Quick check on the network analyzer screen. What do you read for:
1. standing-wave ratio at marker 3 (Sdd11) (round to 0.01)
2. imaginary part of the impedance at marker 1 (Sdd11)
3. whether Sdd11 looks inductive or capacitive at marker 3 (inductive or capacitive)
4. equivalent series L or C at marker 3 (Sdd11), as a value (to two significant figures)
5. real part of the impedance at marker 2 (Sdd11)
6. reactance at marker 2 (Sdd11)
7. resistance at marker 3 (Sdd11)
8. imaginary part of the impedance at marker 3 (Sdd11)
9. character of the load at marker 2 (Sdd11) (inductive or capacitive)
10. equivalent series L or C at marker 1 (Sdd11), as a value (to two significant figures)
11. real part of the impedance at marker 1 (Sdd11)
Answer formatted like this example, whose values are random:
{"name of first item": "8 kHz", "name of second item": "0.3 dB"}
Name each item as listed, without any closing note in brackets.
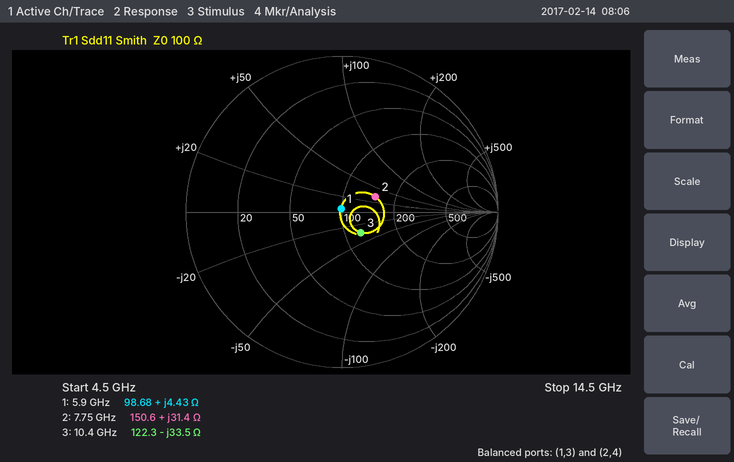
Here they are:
{"standing-wave ratio at marker 3 (Sdd11)": "1.44", "imaginary part of the impedance at marker 1": "+4.43 Ω", "whether Sdd11 looks inductive or capacitive at marker 3": "capacitive", "equivalent series L or C at marker 3 (Sdd11), as a value": "460 fF", "real part of the impedance at marker 2": "150.6 Ω", "reactance at marker 2": "+31.4 Ω", "resistance at marker 3": "122.3 Ω", "imaginary part of the impedance at marker 3": "-33.5 Ω", "character of the load at marker 2 (Sdd11)": "inductive", "equivalent series L or C at marker 1 (Sdd11), as a value": "120 pH", "real part of the impedance at marker 1": "98.68 Ω"}
